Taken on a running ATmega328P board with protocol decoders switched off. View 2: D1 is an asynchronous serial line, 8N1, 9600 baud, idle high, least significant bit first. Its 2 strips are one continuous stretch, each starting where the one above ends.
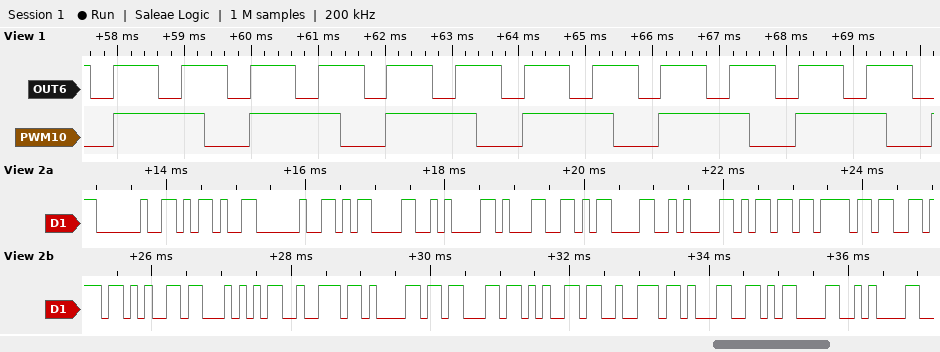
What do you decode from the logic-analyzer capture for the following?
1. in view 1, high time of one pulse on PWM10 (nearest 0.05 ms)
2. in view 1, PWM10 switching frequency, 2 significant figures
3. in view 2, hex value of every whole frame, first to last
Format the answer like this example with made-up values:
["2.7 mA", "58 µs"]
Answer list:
["1.35 ms", "490 Hz", "20 2D 20 0D 0A 31 0D 0A 6D 6F 76 65 54 72 61 63 65 72 31 0D 0A"]
